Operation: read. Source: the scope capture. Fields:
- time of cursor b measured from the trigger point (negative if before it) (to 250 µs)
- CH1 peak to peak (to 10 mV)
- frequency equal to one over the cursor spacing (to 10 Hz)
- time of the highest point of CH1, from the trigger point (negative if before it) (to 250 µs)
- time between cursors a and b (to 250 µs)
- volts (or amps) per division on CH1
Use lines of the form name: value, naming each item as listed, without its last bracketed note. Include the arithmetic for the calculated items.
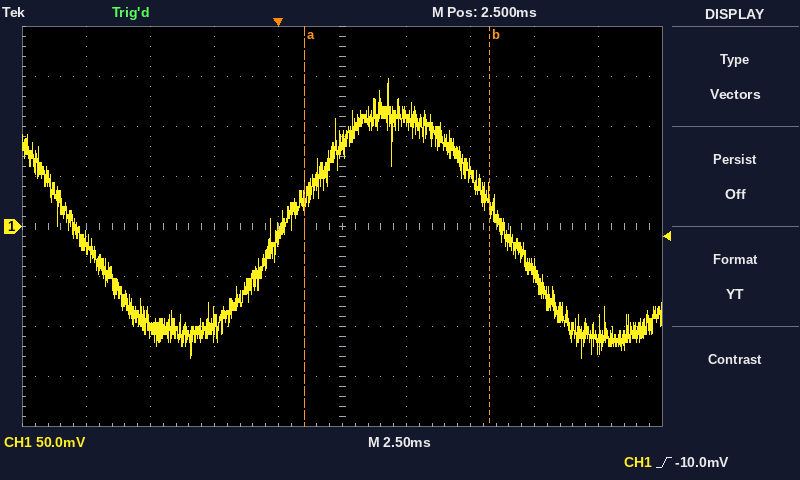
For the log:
time of cursor b measured from the trigger point (negative if before it): +8.25 ms
CH1 peak to peak: 280 mV
frequency equal to one over the cursor spacing: 1 / 7.25 ms ≈ 140 Hz
time of the highest point of CH1, from the trigger point (negative if before it): +4.25 ms
time between cursors a and b: 7.25 ms
volts (or amps) per division on CH1: 50 mV
